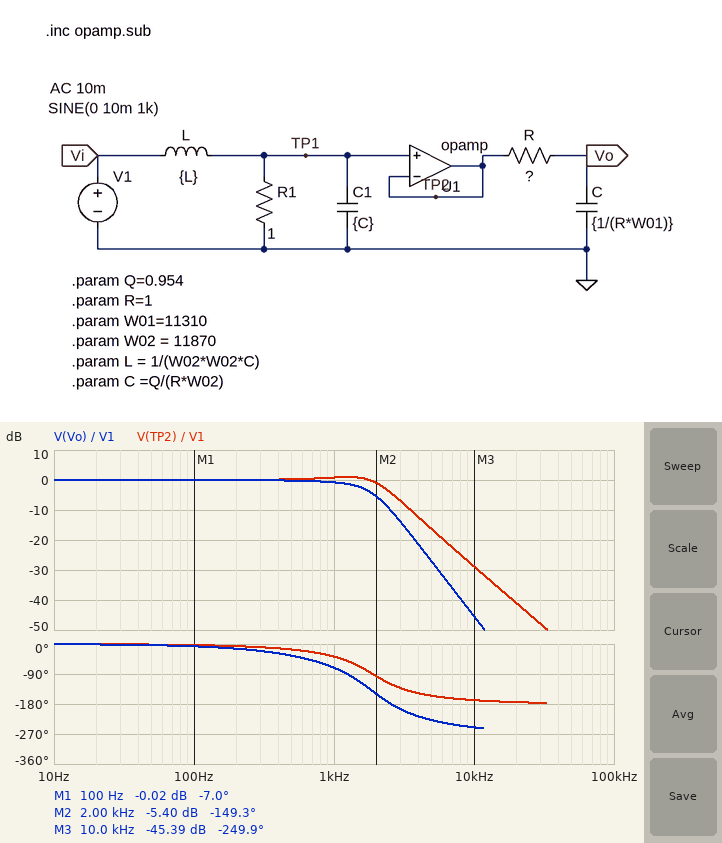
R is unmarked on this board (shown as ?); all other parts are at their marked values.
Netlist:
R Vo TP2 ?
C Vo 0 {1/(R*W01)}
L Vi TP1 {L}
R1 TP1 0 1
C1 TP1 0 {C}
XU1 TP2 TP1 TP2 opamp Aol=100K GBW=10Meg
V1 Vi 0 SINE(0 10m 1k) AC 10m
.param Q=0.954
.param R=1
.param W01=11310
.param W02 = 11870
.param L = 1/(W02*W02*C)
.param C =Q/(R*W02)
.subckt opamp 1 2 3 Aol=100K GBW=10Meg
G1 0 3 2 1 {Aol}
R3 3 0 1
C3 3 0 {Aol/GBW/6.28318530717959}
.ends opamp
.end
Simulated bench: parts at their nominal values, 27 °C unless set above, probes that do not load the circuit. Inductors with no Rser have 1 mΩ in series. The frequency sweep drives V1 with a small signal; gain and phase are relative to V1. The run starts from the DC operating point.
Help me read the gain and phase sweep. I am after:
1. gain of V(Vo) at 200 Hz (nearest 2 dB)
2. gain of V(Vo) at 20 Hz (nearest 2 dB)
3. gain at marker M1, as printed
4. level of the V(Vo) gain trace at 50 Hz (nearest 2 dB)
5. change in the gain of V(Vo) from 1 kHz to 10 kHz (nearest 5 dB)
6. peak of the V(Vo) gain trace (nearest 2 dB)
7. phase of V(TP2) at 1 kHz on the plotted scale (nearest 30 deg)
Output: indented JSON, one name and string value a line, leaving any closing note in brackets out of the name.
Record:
{
  "gain of V(Vo) at 200 Hz": "0 dB",
  "gain of V(Vo) at 20 Hz": "0 dB",
  "gain at marker M1, as printed": "-0.02 dB",
  "level of the V(Vo) gain trace at 50 Hz": "0 dB",
  "change in the gain of V(Vo) from 1 kHz to 10 kHz": "-45 dB",
  "peak of the V(Vo) gain trace": "0 dB",
  "phase of V(TP2) at 1 kHz on the plotted scale": "-30 deg"
}
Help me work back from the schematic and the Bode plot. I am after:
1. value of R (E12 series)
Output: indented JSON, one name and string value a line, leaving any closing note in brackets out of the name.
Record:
{
  "value of R": "1.2 Ω"
}
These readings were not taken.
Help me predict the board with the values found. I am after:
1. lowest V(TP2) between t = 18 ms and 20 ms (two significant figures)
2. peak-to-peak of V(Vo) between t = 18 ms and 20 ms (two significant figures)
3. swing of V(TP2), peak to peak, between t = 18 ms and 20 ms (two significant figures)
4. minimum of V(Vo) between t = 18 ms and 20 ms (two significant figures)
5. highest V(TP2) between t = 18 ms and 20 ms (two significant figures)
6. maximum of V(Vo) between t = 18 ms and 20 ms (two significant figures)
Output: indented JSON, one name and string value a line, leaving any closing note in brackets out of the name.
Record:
{
  "lowest V(TP2) between t = 18 ms and 20 ms": "-11 mV",
  "peak-to-peak of V(Vo) between t = 18 ms and 20 ms": "18 mV",
  "swing of V(TP2), peak to peak, between t = 18 ms and 20 ms": "22 mV",
  "minimum of V(Vo) between t = 18 ms and 20 ms": "-9.1 mV",
  "highest V(TP2) between t = 18 ms and 20 ms": "11 mV",
  "maximum of V(Vo) between t = 18 ms and 20 ms": "9.1 mV"
}
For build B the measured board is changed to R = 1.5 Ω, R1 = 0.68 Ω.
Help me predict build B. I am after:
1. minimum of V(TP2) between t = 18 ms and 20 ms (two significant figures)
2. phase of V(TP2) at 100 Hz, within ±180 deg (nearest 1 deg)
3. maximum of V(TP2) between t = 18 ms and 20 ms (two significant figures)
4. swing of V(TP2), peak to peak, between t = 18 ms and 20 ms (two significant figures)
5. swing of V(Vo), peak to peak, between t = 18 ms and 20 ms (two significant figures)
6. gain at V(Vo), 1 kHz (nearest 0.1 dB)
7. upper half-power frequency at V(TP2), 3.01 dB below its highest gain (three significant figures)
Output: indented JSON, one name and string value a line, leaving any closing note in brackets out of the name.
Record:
{
  "minimum of V(TP2) between t = 18 ms and 20 ms": "-9.2 mV",
  "phase of V(TP2) at 100 Hz, within ±180 deg": "-5 deg",
  "maximum of V(TP2) between t = 18 ms and 20 ms": "9.2 mV",
  "swing of V(TP2), peak to peak, between t = 18 ms and 20 ms": "18 mV",
  "swing of V(Vo), peak to peak, between t = 18 ms and 20 ms": "14 mV",
  "gain at V(Vo), 1 kHz": "-3.0 dB",
  "upper half-power frequency at V(TP2), 3.01 dB below its highest gain": "1.72 kHz"
}
